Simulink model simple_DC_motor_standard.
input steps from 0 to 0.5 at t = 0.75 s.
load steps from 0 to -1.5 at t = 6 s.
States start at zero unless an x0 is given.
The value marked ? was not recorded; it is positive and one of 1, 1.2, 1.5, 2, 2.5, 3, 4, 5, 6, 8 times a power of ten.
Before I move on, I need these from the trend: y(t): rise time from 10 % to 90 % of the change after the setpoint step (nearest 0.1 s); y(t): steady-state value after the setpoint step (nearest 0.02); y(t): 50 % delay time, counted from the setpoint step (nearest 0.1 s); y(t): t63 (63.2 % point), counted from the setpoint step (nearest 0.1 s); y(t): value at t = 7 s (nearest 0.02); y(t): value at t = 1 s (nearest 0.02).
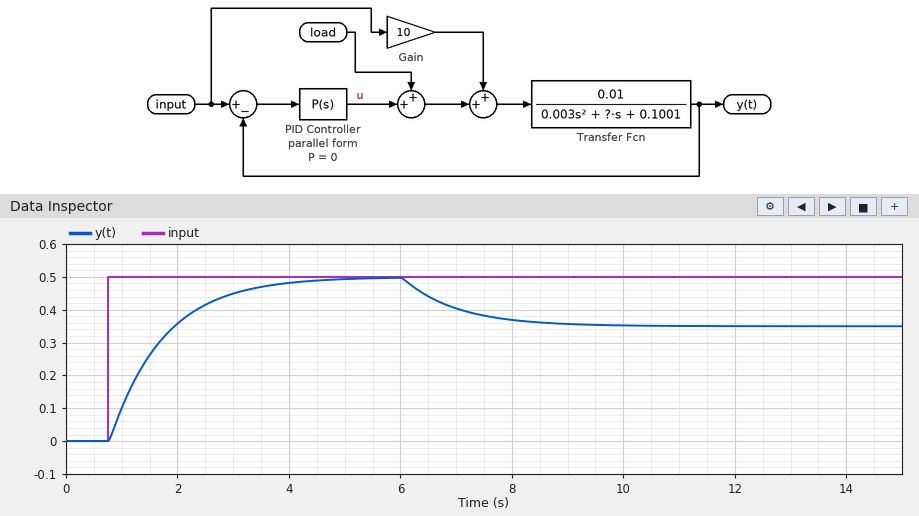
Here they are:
2.1 s
0.50
0.7 s
1.0 s
0.40
0.10
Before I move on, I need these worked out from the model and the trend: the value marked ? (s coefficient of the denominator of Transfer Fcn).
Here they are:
0.1
